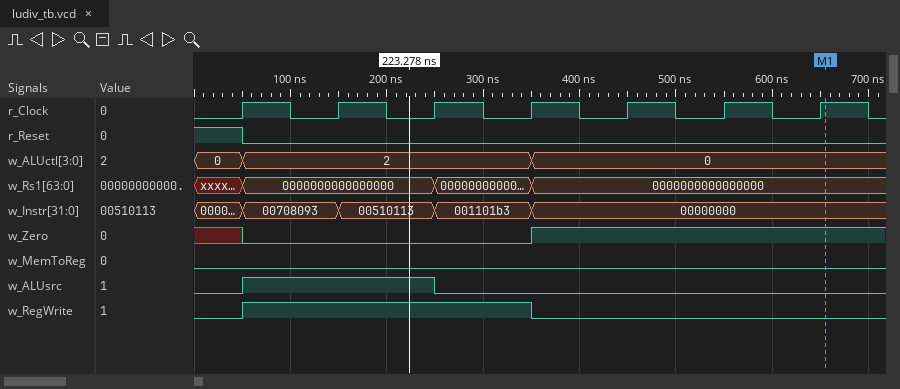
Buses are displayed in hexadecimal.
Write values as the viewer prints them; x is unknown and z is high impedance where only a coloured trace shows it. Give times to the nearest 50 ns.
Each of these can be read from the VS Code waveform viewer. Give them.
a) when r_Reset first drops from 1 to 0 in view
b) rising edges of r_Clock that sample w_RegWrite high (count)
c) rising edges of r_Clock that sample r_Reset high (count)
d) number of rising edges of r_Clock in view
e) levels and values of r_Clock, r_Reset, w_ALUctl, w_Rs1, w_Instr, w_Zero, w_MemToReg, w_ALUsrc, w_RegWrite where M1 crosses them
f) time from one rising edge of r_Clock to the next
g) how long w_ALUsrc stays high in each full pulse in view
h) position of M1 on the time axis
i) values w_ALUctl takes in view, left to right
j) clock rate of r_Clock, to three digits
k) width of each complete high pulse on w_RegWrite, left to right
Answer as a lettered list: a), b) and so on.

a) 50 ns
b) 3
c) 1
d) 7
e) r_Clock=1, r_Reset=0, w_ALUctl=0, w_Rs1=0000000000000000, w_Instr=00000000, w_Zero=1, w_MemToReg=0, w_ALUsrc=0, w_RegWrite=0
f) 100 ns
g) 200 ns
h) 650 ns
i) 0, 2, 0
j) 10.0 MHz
k) 300 ns
